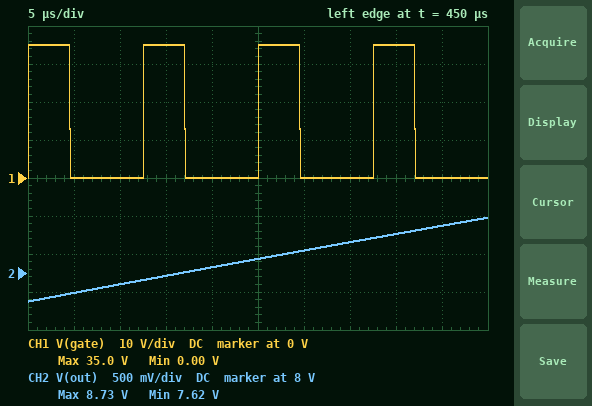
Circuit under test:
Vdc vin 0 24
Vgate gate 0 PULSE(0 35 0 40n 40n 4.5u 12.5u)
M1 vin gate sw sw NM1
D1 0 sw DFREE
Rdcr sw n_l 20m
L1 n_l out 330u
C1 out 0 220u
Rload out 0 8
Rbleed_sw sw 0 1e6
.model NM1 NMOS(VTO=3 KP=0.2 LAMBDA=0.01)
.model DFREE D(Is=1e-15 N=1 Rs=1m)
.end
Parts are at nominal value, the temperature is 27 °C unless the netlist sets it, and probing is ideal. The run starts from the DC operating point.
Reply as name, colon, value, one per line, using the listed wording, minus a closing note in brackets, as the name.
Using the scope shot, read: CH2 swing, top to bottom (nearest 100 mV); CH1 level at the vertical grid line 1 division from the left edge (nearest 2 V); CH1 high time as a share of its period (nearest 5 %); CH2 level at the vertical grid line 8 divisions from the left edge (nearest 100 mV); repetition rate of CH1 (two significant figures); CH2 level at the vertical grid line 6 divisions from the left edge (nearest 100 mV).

CH2 swing, top to bottom: 1.1 V
CH1 level at the vertical grid line 1 division from the left edge: 0 V
CH1 high time as a share of its period: 35 %
CH2 level at the vertical grid line 8 divisions from the left edge: 8.5 V
repetition rate of CH1: 80 kHz
CH2 level at the vertical grid line 6 divisions from the left edge: 8.3 V
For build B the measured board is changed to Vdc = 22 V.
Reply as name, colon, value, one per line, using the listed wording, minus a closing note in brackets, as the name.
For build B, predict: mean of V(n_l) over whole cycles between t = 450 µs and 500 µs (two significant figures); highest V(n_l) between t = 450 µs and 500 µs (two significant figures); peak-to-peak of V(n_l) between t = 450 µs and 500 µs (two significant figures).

mean of V(n_l) over whole cycles between t = 450 µs and 500 µs: 6.4 V
highest V(n_l) between t = 450 µs and 500 µs: 20 V
peak-to-peak of V(n_l) between t = 450 µs and 500 µs: 21 V
